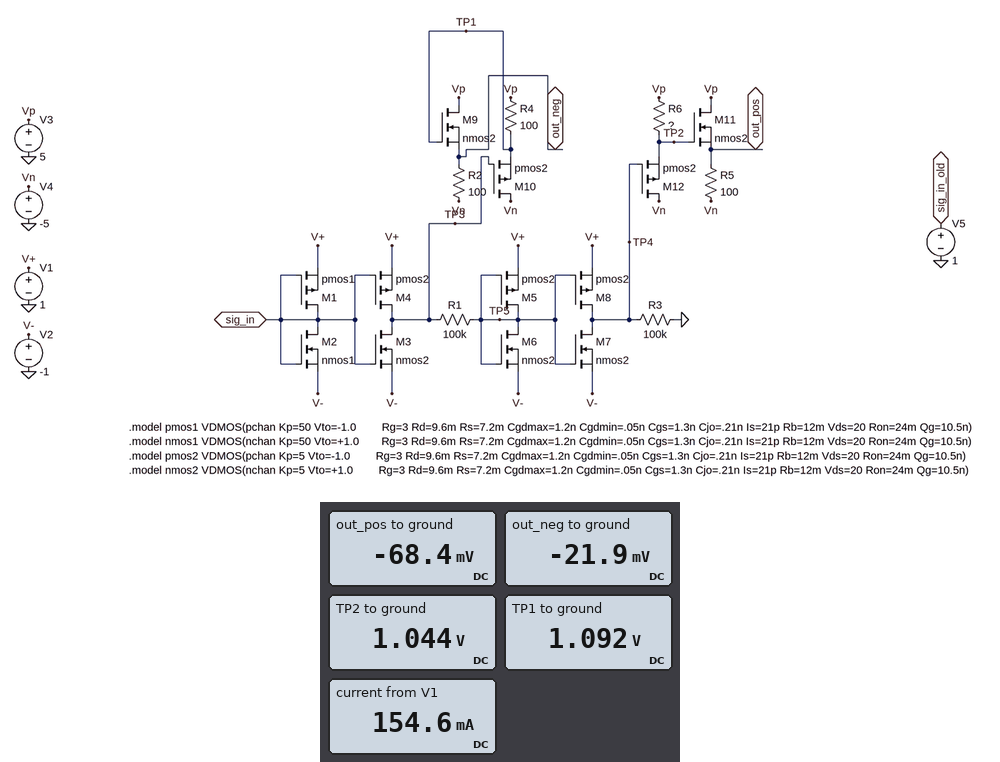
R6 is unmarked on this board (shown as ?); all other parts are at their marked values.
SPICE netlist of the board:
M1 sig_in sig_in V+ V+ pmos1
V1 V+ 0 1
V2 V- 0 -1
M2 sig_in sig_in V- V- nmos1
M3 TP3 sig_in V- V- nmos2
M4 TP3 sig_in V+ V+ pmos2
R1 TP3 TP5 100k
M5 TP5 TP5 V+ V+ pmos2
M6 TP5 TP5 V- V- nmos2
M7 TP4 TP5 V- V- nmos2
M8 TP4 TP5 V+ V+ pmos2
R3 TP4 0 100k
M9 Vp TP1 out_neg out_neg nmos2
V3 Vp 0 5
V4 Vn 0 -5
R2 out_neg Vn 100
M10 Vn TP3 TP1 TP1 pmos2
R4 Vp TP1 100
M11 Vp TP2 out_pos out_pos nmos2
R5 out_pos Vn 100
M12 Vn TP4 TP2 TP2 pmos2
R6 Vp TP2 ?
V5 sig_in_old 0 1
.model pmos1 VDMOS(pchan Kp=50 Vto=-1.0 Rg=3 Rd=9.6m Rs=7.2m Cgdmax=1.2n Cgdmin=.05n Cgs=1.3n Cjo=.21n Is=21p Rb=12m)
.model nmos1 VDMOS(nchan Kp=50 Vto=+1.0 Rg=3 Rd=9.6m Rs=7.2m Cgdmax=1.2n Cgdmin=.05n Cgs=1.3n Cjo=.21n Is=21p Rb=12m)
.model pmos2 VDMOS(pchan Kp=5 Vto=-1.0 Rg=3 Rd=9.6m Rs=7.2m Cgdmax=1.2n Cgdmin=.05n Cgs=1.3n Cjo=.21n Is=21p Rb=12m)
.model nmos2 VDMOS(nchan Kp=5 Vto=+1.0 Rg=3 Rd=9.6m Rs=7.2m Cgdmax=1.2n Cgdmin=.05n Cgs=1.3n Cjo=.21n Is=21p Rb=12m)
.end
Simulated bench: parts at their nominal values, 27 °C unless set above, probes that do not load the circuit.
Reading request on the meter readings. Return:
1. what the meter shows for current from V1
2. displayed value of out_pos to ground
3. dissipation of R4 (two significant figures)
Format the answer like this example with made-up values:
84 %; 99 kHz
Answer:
154.6 mA; -68.4 mV; 150 mW
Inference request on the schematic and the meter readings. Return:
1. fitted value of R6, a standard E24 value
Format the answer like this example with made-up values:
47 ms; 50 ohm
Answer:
180 Ω
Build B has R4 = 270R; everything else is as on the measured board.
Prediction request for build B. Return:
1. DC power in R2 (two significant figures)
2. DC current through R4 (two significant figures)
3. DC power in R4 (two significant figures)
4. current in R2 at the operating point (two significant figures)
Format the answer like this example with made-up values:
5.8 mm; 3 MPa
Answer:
240 mW; 15 mA; 59 mW; 49 mA
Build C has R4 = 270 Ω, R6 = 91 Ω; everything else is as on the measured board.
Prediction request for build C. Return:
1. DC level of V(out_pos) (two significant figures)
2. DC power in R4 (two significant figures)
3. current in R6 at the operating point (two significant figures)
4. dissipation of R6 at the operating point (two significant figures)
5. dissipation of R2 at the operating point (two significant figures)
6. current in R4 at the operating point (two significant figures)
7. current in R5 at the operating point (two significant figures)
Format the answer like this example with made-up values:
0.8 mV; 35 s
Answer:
-14 mV; 59 mW; 43 mA; 170 mW; 240 mW; 15 mA; 50 mA
